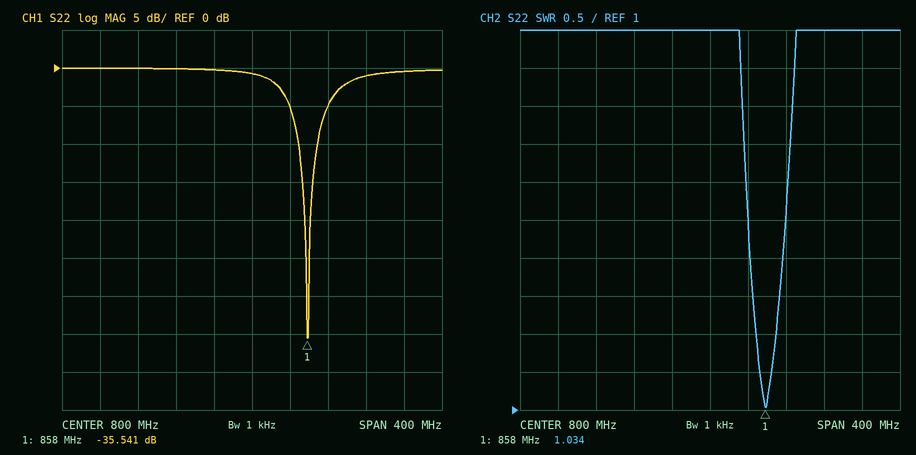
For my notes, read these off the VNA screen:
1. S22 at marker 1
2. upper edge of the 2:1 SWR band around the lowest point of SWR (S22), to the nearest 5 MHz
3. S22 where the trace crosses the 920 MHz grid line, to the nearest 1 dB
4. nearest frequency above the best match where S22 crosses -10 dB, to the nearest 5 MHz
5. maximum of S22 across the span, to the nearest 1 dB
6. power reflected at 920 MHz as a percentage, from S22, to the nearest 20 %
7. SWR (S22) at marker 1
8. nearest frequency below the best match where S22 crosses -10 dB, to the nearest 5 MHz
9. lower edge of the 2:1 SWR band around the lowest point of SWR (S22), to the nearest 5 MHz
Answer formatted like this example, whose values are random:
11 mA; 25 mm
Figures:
-35.541 dB; 870 MHz; -1 dB; 870 MHz; 0 dB; 80 %; 1.034; 850 MHz; 850 MHz
